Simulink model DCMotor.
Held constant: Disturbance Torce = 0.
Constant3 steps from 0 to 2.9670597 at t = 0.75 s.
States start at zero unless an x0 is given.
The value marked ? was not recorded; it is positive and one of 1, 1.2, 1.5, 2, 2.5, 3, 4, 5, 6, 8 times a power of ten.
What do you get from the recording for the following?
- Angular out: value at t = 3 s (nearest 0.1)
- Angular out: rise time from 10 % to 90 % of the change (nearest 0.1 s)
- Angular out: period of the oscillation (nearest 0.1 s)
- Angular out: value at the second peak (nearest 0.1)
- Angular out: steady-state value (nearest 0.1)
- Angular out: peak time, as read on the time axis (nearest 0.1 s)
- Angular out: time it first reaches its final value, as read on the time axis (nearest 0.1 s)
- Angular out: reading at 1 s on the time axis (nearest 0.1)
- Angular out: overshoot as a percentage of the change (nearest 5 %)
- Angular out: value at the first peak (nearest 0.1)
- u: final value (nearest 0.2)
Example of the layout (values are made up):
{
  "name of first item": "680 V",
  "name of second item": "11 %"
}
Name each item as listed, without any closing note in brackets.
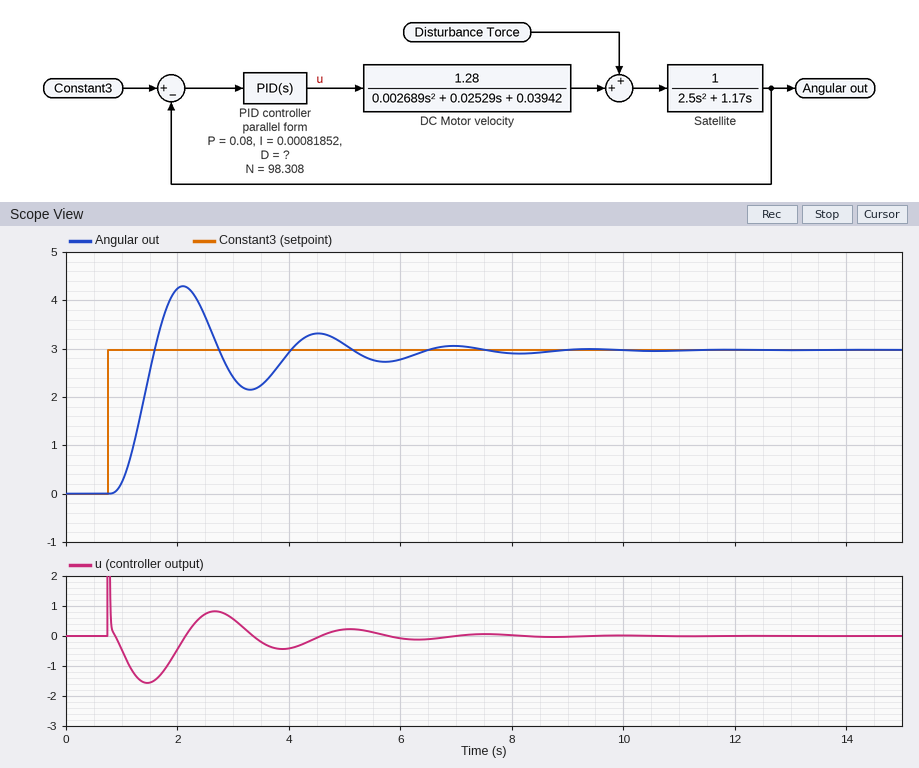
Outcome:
{
  "Angular out: value at t = 3 s": "2.4",
  "Angular out: rise time from 10 % to 90 % of the change": "0.5 s",
  "Angular out: period of the oscillation": "2.4 s",
  "Angular out: value at the second peak": "3.3",
  "Angular out: steady-state value": "3.0",
  "Angular out: peak time, as read on the time axis": "2.1 s",
  "Angular out: time it first reaches its final value, as read on the time axis": "1.6 s",
  "Angular out: reading at 1 s on the time axis": "0.2",
  "Angular out: overshoot as a percentage of the change": "45 %",
  "Angular out: value at the first peak": "4.3",
  "u: final value": "0.0"
}
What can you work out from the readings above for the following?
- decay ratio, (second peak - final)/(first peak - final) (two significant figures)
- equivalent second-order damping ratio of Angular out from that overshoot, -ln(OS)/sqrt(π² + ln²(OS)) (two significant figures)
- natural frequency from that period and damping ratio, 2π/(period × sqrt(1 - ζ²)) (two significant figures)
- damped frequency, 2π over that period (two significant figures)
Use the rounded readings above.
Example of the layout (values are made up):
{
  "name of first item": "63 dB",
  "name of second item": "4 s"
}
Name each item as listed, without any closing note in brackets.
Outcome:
{
  "decay ratio, (second peak - final)/(first peak - final)": "0.23",
  "equivalent second-order damping ratio of Angular out from that overshoot, -ln(OS)/sqrt(π² + ln²(OS))": "0.25",
  "natural frequency from that period and damping ratio, 2π/(period × sqrt(1 - ζ²))": "2.7 rad/s",
  "damped frequency, 2π over that period": "2.6 rad/s"
}
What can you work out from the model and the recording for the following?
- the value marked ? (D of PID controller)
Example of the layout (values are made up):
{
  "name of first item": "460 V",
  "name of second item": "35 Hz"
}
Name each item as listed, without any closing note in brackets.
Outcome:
{
  "the value marked ?": "0.3"
}
